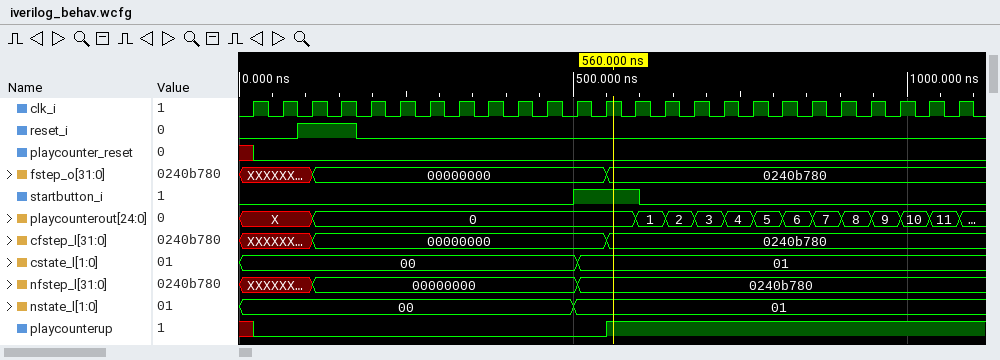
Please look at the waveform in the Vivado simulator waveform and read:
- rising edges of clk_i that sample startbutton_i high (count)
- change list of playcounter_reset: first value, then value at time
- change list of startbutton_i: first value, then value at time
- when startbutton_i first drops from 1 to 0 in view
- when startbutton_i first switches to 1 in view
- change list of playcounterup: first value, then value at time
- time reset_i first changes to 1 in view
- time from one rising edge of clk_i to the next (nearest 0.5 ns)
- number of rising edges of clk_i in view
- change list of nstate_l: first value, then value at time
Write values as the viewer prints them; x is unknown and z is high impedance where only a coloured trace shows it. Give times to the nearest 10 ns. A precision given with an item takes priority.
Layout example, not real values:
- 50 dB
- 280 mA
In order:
- 3
- x, 0 at 20 ns
- 0, 1 at 500 ns, 0 at 600 ns
- 600 ns
- 500 ns
- x, 0 at 20 ns, 1 at 550 ns
- 90 ns
- 44 ns
- 25
- 00, 01 at 500 ns
